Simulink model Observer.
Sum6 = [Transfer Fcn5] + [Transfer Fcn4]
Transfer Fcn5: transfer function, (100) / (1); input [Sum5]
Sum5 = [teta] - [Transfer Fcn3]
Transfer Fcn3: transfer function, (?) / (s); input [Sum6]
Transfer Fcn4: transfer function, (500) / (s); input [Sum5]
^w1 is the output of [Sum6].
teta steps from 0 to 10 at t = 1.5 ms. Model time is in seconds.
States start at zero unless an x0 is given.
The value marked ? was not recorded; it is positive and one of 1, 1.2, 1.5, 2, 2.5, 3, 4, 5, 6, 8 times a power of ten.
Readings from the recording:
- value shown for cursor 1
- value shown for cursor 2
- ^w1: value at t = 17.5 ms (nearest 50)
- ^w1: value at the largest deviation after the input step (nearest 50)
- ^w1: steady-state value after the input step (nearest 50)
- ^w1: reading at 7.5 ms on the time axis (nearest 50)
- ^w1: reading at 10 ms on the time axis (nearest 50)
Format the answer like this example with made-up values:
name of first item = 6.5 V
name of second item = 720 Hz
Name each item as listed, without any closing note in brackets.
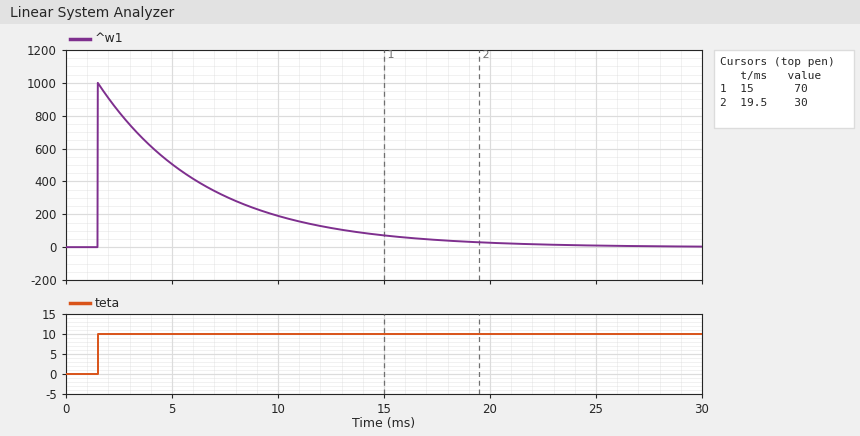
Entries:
value shown for cursor 1 = 70
value shown for cursor 2 = 30
^w1: value at t = 17.5 ms = 50
^w1: value at the largest deviation after the input step = 1000
^w1: steady-state value after the input step = 0
^w1: reading at 7.5 ms on the time axis = 300
^w1: reading at 10 ms on the time axis = 200
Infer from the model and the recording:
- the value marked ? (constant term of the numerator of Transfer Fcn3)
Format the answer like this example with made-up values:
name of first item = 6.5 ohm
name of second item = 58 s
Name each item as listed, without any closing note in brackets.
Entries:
the value marked ? = 2
